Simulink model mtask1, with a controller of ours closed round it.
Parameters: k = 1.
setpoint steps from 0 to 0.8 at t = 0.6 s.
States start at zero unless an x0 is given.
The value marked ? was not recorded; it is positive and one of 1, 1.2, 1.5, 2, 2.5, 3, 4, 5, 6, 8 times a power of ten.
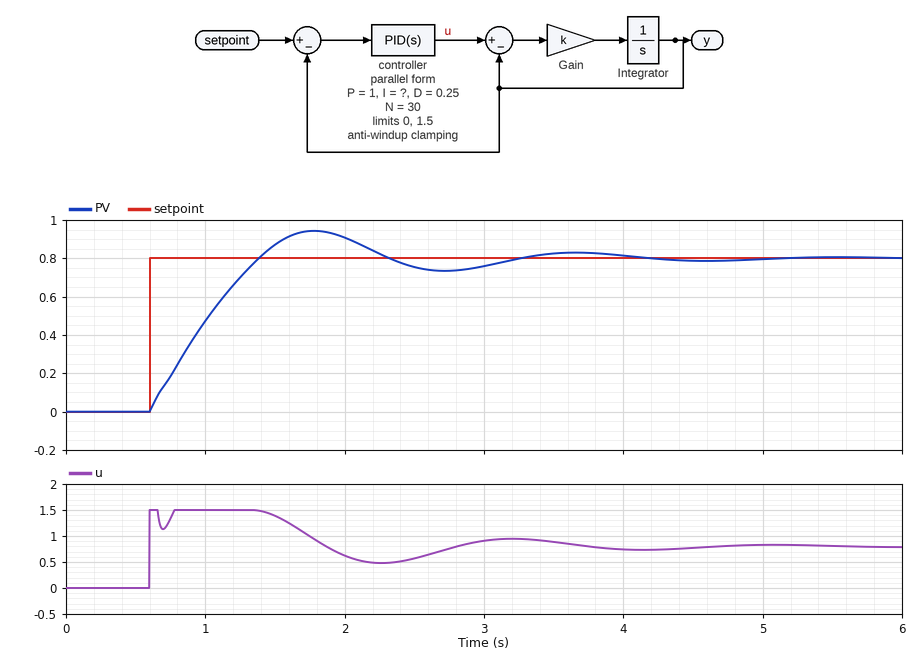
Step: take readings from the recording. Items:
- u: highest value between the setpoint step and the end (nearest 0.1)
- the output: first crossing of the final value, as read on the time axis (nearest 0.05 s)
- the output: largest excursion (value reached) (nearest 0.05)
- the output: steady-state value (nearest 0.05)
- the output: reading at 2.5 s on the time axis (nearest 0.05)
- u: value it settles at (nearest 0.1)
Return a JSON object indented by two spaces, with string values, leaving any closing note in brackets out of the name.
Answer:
{
  "u: highest value between the setpoint step and the end": "1.5",
  "the output: first crossing of the final value, as read on the time axis": "1.40 s",
  "the output: largest excursion (value reached)": "0.95",
  "the output: steady-state value": "0.80",
  "the output: reading at 2.5 s on the time axis": "0.75",
  "u: value it settles at": "0.8"
}
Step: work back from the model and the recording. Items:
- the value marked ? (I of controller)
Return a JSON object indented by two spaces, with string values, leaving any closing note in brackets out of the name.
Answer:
{
  "the value marked ?": "15"
}
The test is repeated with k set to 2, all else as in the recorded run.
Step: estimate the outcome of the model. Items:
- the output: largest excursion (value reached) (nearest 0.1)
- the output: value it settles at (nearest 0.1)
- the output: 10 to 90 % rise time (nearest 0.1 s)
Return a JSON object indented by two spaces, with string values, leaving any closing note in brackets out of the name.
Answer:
{
  "the output: largest excursion (value reached)": "1.0",
  "the output: value it settles at": "0.8",
  "the output: 10 to 90 % rise time": "0.4 s"
}
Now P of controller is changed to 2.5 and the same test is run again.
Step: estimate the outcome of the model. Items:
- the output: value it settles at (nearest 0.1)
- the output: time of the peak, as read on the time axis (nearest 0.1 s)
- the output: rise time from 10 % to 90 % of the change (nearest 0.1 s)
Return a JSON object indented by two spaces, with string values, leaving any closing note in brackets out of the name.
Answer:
{
  "the output: value it settles at": "0.8",
  "the output: time of the peak, as read on the time axis": "1.7 s",
  "the output: rise time from 10 % to 90 % of the change": "0.6 s"
}
